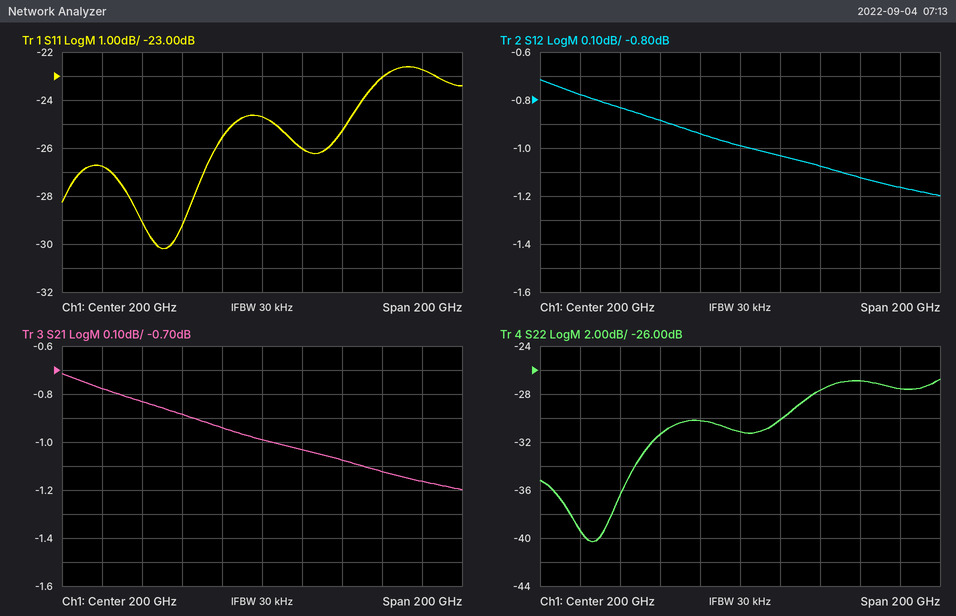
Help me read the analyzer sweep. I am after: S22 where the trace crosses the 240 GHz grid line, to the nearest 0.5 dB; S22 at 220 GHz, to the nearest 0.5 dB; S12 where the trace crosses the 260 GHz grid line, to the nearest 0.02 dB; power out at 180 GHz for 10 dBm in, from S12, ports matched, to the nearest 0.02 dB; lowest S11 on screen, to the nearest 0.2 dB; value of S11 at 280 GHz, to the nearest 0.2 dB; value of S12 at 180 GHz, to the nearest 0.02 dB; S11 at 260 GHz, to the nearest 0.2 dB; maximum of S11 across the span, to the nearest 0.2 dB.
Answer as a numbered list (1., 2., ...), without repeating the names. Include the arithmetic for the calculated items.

1. -27.5 dB
2. -30.0 dB
3. -1.12 dB
4. 10 dBm + (-0.94 dB) = 9.06 dBm
5. -30.2 dB
6. -22.8 dB
7. -0.94 dB
8. -23.0 dB
9. -22.6 dB
